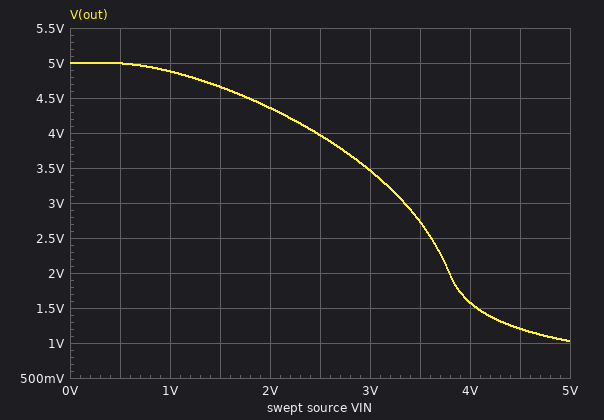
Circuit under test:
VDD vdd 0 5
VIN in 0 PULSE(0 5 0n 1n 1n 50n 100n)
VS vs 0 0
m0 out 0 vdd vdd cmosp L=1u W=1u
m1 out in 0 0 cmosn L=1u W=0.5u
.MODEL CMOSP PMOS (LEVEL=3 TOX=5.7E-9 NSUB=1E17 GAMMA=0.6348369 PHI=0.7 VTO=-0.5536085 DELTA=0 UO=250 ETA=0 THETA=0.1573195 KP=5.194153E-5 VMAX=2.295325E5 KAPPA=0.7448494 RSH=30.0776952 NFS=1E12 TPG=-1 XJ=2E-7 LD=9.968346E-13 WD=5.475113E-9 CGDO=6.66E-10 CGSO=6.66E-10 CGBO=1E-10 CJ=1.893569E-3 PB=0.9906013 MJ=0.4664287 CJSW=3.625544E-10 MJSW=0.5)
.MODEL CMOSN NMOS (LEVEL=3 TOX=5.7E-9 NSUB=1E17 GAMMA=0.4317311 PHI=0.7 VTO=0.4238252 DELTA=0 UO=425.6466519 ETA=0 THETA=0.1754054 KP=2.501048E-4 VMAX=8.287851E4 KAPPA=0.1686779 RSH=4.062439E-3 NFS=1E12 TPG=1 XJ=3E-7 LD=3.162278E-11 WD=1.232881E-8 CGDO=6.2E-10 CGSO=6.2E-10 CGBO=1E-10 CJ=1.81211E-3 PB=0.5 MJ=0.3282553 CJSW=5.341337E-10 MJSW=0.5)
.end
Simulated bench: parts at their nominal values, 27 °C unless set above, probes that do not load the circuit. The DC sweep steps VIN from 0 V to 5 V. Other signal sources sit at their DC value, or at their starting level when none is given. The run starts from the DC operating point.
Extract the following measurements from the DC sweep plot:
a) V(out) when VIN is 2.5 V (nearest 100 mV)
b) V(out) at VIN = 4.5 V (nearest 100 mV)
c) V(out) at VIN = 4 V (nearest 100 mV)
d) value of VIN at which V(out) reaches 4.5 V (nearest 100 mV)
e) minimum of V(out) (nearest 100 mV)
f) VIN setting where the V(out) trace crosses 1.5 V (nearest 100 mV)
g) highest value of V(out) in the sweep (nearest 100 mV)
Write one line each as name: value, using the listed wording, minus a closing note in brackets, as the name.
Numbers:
V(out) when VIN is 2.5 V: 4.0 V
V(out) at VIN = 4.5 V: 1.2 V
V(out) at VIN = 4 V: 1.6 V
value of VIN at which V(out) reaches 4.5 V: 1.8 V
minimum of V(out): 1.0 V
VIN setting where the V(out) trace crosses 1.5 V: 4.1 V
highest value of V(out) in the sweep: 5.0 V
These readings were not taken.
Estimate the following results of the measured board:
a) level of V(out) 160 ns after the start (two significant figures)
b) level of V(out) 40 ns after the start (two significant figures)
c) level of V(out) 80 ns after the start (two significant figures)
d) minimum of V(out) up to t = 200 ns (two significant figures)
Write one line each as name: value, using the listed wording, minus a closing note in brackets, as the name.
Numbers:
level of V(out) 160 ns after the start: 5.0 V
level of V(out) 40 ns after the start: 1.0 V
level of V(out) 80 ns after the start: 5.0 V
minimum of V(out) up to t = 200 ns: 1.0 V
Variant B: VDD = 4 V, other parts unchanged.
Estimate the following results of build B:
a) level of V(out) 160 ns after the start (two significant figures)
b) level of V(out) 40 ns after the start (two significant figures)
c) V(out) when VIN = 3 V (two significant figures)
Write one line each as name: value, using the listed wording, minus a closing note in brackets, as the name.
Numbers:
level of V(out) 160 ns after the start: 4.0 V
level of V(out) 40 ns after the start: 600 mV
V(out) when VIN = 3 V: 1.5 V
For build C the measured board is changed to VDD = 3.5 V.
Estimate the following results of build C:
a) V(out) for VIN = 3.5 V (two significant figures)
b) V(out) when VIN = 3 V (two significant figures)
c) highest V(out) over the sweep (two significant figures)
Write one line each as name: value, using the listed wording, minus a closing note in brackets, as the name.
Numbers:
V(out) for VIN = 3.5 V: 650 mV
V(out) when VIN = 3 V: 840 mV
highest V(out) over the sweep: 3.5 V
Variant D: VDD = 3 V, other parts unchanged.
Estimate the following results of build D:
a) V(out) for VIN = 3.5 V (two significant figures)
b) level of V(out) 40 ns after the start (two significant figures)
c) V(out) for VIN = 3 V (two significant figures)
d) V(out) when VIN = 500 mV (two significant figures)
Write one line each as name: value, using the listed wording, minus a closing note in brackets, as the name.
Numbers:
V(out) for VIN = 3.5 V: 440 mV
level of V(out) 40 ns after the start: 320 mV
V(out) for VIN = 3 V: 530 mV
V(out) when VIN = 500 mV: 3.0 V
